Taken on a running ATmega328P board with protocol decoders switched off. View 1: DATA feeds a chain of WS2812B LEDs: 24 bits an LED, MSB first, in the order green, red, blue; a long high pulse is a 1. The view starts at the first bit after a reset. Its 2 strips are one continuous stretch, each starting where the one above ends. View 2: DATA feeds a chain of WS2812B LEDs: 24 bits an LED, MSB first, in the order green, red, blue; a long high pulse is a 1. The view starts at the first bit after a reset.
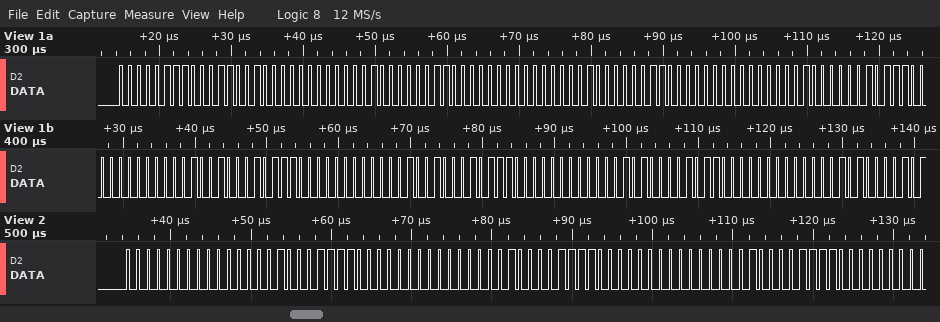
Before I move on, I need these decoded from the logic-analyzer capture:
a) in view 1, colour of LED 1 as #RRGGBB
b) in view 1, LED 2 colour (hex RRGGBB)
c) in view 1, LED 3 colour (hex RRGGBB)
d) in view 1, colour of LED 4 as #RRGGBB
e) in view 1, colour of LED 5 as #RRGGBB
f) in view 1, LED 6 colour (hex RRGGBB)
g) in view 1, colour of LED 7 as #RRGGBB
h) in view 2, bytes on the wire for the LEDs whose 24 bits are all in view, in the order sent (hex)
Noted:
#190700
#180800
#180800
#170800
#170900
#170900
#160A00
00 01 1E 00 02 1E 00 02 1E
